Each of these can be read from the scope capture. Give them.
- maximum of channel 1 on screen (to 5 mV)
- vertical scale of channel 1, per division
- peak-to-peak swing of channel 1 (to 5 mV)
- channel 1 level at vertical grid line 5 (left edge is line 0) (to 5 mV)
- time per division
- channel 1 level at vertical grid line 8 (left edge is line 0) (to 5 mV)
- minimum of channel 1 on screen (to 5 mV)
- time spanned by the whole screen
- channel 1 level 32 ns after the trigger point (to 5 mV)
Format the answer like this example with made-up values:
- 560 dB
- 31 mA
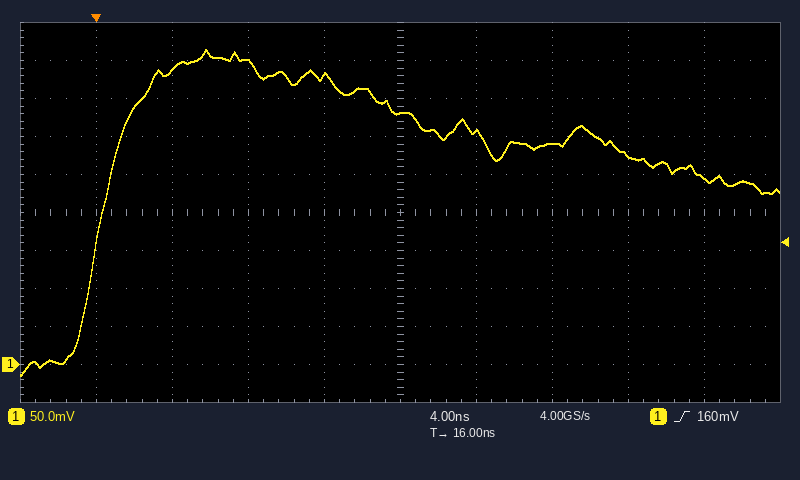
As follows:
- 415 mV
- 50 mV
- 430 mV
- 330 mV
- 4 ns
- 275 mV
- -15 mV
- 40 ns
- 245 mV
